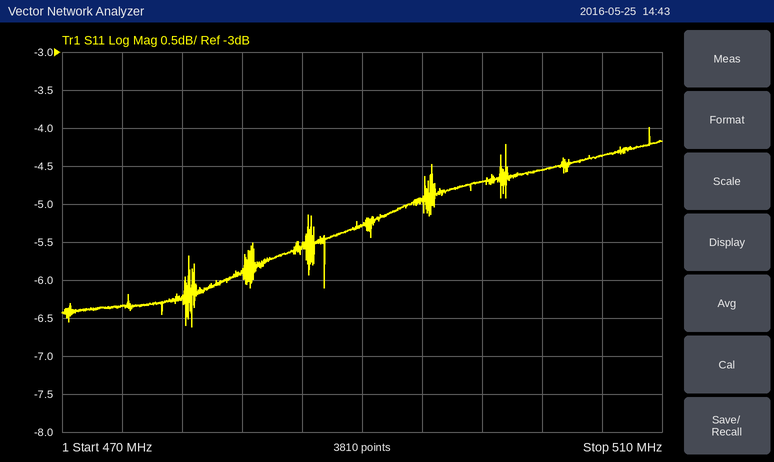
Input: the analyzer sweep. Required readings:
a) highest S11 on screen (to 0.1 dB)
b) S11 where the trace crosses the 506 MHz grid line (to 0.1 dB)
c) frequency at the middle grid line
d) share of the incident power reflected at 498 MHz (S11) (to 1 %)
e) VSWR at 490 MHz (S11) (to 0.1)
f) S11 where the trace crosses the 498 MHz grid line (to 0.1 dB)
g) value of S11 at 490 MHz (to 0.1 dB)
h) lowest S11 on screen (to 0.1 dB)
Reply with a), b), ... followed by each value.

a) -4.0 dB
b) -4.4 dB
c) 490 MHz
d) 34 %
e) 3.4
f) -4.7 dB
g) -5.3 dB
h) -6.6 dB
